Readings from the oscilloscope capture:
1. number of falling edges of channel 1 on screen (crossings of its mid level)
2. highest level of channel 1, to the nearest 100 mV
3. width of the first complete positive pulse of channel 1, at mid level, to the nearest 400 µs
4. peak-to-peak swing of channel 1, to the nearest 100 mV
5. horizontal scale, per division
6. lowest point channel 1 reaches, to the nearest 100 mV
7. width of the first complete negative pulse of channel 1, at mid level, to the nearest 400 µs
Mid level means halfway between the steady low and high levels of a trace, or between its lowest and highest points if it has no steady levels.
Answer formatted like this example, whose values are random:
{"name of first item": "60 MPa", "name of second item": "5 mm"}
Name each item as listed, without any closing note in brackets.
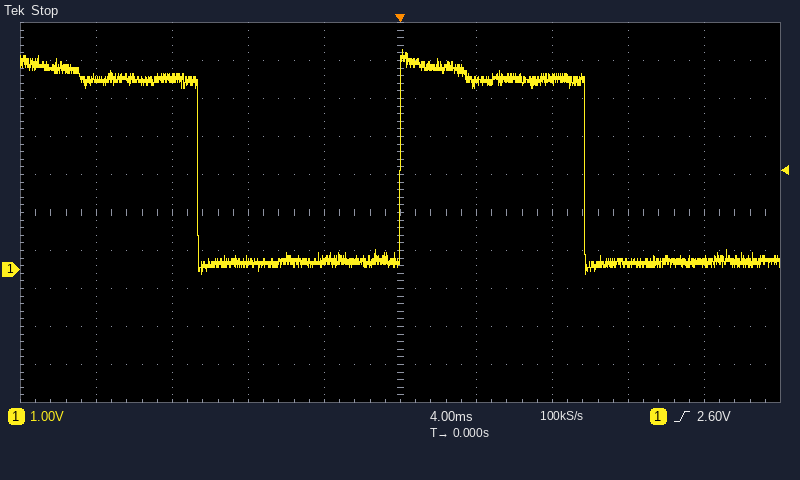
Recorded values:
{"number of falling edges of channel 1 on screen": "2", "highest level of channel 1, to the nearest 100 mV": "5.8 V", "width of the first complete positive pulse of channel 1, at mid level, to the nearest 400 µs": "9.6 ms", "peak-to-peak swing of channel 1, to the nearest 100 mV": "5.9 V", "horizontal scale, per division": "4 ms", "lowest point channel 1 reaches, to the nearest 100 mV": "-100 mV", "width of the first complete negative pulse of channel 1, at mid level, to the nearest 400 µs": "10.8 ms"}
